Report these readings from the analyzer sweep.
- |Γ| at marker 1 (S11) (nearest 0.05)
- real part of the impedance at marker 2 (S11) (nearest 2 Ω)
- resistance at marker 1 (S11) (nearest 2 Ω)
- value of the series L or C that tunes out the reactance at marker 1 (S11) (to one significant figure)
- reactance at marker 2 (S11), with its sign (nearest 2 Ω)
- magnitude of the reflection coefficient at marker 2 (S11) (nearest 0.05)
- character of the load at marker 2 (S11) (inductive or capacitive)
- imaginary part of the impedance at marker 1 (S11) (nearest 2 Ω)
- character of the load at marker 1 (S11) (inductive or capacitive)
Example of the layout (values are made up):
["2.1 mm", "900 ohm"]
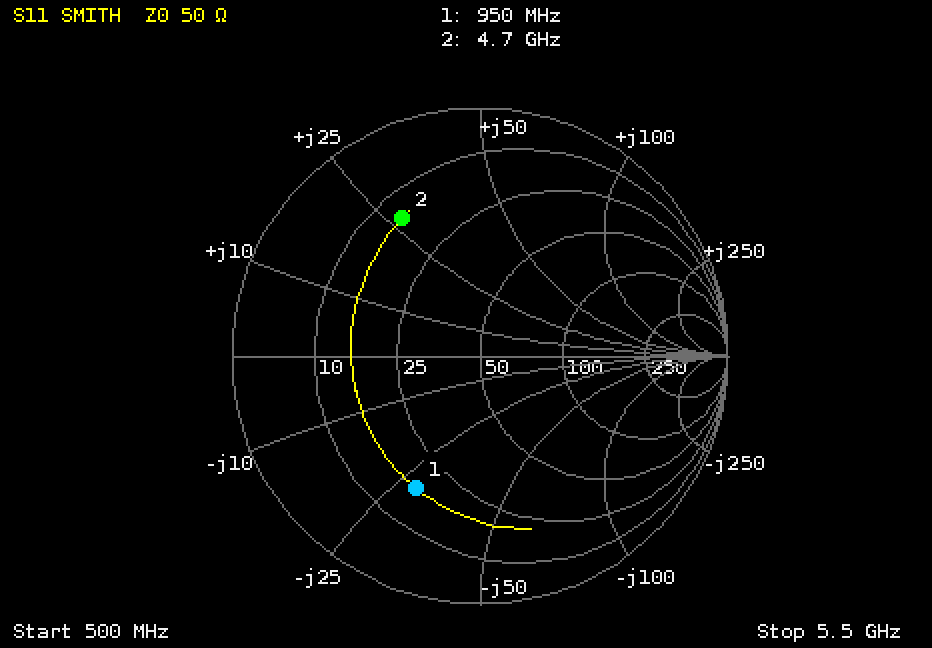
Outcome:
["0.60", "14 Ω", "18 Ω", "5 nH", "+28 Ω", "0.65", "inductive", "-28 Ω", "capacitive"]
